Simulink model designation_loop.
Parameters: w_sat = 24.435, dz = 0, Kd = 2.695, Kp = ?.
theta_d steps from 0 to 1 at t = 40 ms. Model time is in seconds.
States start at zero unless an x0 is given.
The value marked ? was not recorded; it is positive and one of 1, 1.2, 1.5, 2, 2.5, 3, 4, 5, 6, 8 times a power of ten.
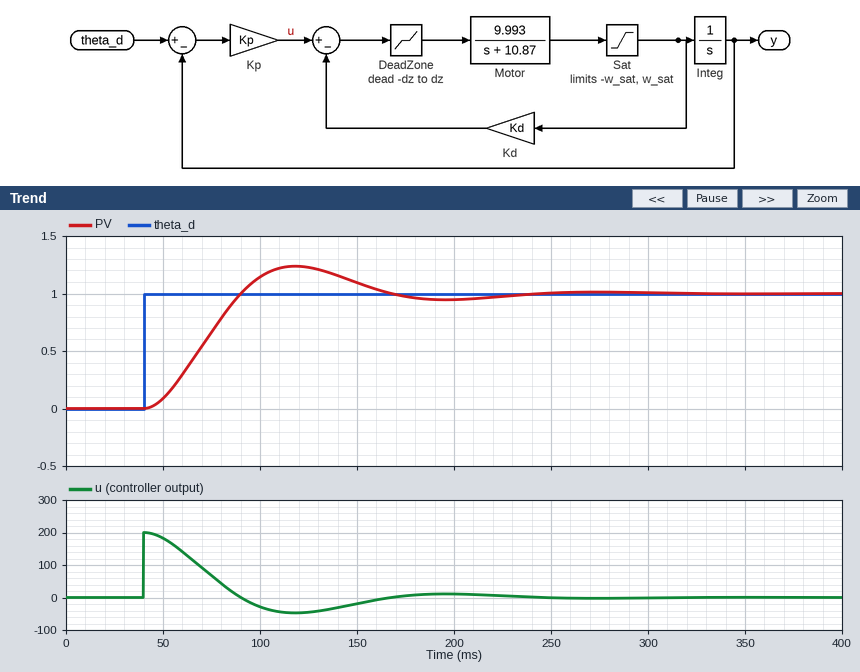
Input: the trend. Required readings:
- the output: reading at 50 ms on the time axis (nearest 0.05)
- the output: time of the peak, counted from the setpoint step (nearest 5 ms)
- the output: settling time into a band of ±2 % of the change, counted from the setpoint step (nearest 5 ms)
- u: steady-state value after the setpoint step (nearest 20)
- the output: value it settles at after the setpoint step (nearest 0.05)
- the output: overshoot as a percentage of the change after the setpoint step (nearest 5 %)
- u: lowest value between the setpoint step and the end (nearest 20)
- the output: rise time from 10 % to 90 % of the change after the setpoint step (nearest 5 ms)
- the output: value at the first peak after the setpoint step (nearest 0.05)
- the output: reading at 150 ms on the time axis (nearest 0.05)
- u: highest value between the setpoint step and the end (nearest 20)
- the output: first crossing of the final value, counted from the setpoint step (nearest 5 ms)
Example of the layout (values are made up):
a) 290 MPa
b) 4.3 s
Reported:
a) 0.10
b) 80 ms
c) 190 ms
d) 0
e) 1.00
f) 25 %
g) -40
h) 35 ms
i) 1.25
j) 1.10
k) 200
l) 50 ms
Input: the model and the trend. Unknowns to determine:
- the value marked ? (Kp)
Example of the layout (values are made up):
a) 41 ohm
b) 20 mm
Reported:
a) 200
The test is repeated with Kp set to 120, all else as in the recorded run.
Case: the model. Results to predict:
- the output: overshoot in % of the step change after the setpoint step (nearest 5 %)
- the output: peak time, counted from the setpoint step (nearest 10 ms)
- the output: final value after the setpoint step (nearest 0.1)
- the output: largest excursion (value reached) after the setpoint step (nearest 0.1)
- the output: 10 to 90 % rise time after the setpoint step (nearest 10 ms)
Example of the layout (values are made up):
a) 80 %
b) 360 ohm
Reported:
a) 15 %
b) 110 ms
c) 1.0
d) 1.1
e) 50 ms
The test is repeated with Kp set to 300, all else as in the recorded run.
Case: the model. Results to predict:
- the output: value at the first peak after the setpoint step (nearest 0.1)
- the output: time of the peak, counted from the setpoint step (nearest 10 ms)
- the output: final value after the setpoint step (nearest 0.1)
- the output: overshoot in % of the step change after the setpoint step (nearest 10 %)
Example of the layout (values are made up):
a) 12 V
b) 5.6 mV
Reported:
a) 1.4
b) 70 ms
c) 1.0
d) 40 %
